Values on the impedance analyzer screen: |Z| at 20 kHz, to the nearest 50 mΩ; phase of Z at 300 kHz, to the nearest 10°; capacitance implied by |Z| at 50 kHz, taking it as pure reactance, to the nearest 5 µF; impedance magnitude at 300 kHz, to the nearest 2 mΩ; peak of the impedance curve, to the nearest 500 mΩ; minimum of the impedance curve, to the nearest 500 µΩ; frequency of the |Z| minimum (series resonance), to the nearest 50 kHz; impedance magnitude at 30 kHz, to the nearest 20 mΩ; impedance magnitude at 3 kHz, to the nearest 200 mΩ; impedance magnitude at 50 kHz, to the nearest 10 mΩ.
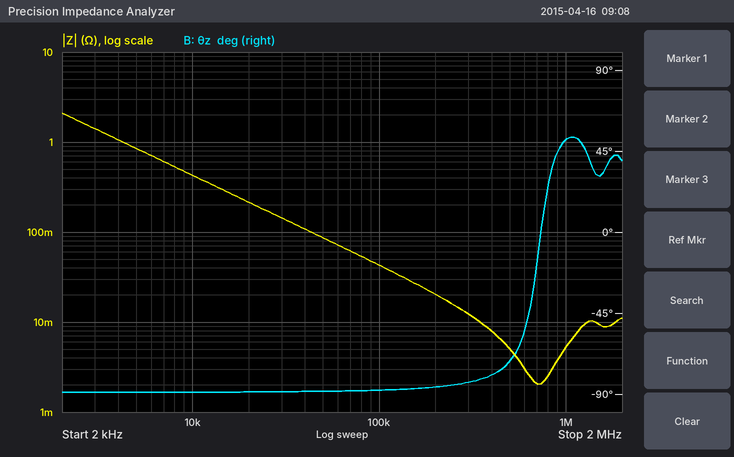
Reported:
200 mΩ
-80°
35 µF
12 mΩ
2.0 Ω
2.0 mΩ
700 kHz
140 mΩ
1.4 Ω
90 mΩ
